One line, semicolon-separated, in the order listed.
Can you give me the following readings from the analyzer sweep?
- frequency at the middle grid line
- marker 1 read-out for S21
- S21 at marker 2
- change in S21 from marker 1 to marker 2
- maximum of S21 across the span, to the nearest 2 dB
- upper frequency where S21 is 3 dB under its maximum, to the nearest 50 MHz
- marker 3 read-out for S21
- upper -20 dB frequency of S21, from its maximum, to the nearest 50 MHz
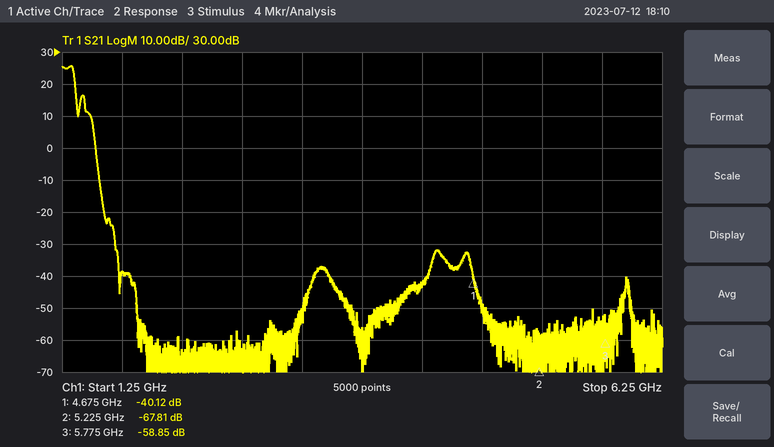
3.75 GHz; -40.12 dB; -67.81 dB; -27.69 dB; 26 dB; 1.35 GHz; -58.85 dB; 1.50 GHz
